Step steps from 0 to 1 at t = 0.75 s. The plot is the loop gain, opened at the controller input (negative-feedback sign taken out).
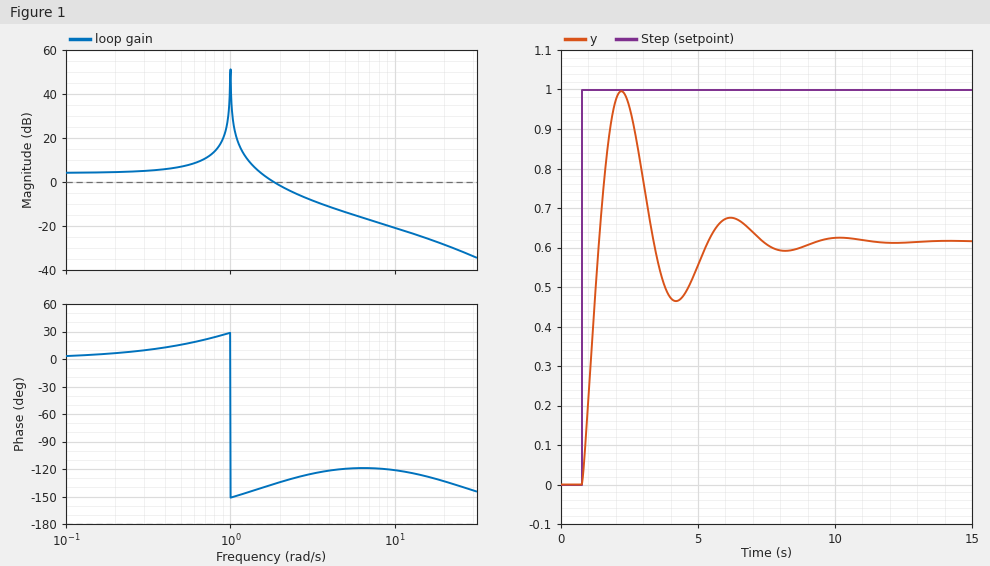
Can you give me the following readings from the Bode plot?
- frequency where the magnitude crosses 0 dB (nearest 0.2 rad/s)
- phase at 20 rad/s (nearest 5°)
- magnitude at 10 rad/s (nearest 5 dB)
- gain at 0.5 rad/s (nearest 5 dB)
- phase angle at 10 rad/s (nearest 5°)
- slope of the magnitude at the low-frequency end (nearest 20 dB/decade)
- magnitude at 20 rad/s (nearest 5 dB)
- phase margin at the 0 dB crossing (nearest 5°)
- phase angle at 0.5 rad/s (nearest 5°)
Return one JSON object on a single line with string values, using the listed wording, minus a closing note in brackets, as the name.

{"frequency where the magnitude crosses 0 dB": "1.8 rad/s", "phase at 20 rad/s": "-135°", "magnitude at 10 rad/s": "-20 dB", "gain at 0.5 rad/s": "5 dB", "phase angle at 10 rad/s": "-120°", "slope of the magnitude at the low-frequency end": "0 dB/decade", "magnitude at 20 rad/s": "-30 dB", "phase margin at the 0 dB crossing": "45°", "phase angle at 0.5 rad/s": "15°"}
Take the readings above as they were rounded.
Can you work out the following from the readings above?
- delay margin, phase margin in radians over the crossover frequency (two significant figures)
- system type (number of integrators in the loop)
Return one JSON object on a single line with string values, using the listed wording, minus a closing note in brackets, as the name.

{"delay margin, phase margin in radians over the crossover frequency": "0.44 s", "system type": "0"}
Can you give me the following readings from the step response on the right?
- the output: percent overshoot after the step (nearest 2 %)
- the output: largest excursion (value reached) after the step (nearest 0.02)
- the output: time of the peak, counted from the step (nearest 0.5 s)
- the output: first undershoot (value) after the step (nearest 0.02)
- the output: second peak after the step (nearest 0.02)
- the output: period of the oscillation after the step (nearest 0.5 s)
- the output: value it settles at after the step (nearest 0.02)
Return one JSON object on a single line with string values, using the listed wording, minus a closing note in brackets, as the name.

{"the output: percent overshoot after the step": "62 %", "the output: largest excursion (value reached) after the step": "1.00", "the output: time of the peak, counted from the step": "1.5 s", "the output: first undershoot (value) after the step": "0.46", "the output: second peak after the step": "0.68", "the output: period of the oscillation after the step": "4.0 s", "the output: value it settles at after the step": "0.62"}
